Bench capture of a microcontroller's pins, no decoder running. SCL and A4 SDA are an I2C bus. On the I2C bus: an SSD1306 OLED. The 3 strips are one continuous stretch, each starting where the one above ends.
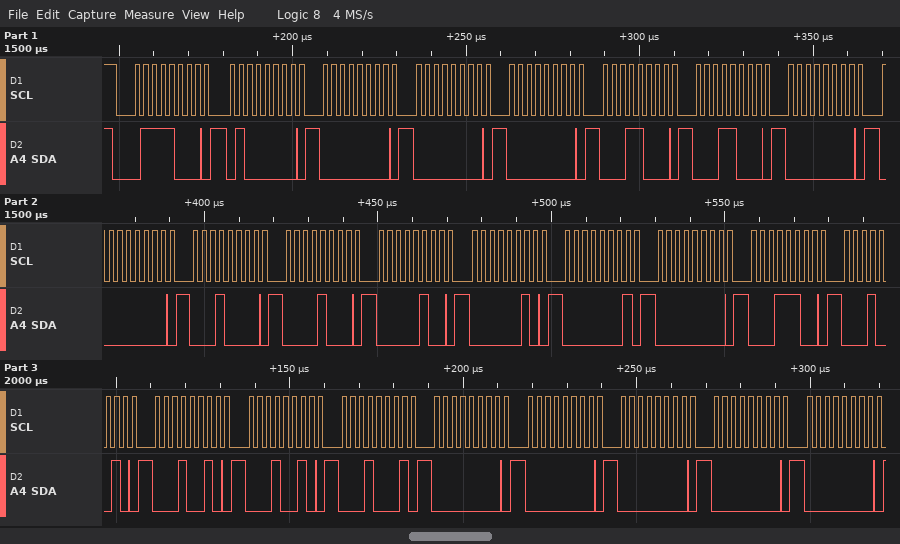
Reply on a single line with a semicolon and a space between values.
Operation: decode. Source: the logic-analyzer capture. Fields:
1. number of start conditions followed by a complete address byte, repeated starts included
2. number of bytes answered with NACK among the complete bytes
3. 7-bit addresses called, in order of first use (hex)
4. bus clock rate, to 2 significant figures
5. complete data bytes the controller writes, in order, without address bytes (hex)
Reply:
1; 0; 0x3C; 400 kHz; 40 00 00 00 18 18 00 00 10 08 04 02 01 00 1C 12 12 12 11 00 00 00 00 00
